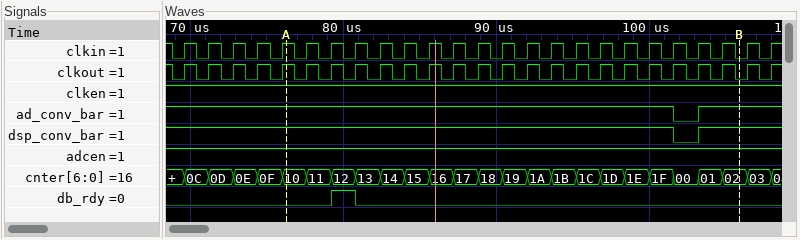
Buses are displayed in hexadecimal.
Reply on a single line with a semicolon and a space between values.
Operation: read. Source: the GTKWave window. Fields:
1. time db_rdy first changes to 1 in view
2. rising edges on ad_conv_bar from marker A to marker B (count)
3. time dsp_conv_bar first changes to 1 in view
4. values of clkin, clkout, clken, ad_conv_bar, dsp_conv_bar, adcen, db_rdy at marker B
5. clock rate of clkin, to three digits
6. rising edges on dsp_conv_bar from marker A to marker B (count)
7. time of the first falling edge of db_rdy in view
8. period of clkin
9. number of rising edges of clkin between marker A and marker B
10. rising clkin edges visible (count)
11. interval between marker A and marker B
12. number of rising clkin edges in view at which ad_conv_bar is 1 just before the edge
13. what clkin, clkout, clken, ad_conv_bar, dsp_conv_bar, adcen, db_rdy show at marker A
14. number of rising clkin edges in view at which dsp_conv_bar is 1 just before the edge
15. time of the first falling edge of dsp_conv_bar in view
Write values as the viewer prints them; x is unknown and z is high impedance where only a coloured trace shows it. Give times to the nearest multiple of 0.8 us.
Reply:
79.2 us; 1; 103.2 us; clkin=0, clkout=0, clken=1, ad_conv_bar=1, dsp_conv_bar=1, adcen=1, db_rdy=0; 625 kHz; 1; 80.8 us; 1.6 us; 18; 25; 29.6 us; 24; clkin=1, clkout=1, clken=1, ad_conv_bar=1, dsp_conv_bar=1, adcen=1, db_rdy=0; 24; 101.6 us
